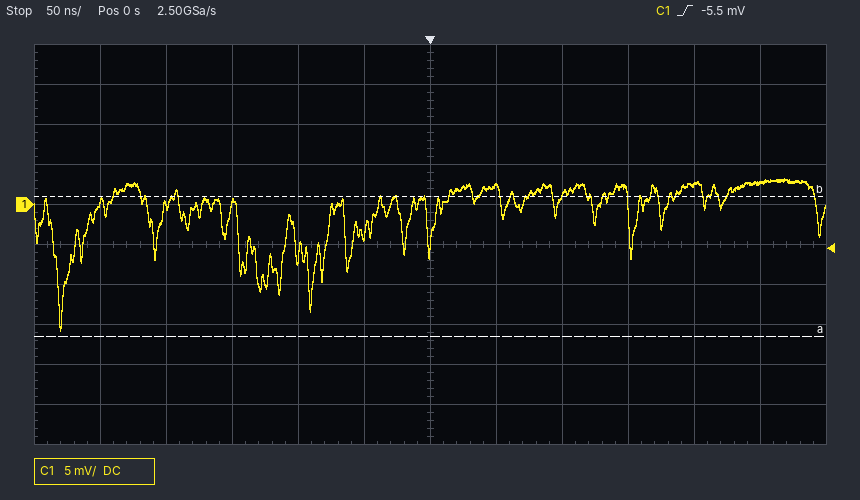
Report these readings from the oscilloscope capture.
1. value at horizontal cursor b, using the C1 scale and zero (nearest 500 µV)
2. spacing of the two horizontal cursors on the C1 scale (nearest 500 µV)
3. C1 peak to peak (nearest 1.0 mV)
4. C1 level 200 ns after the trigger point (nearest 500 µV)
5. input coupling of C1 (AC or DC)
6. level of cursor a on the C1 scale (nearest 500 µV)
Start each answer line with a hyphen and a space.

- 1.0 mV
- 17.5 mV
- 19.0 mV
- 2.5 mV
- DC
- -16.5 mV
